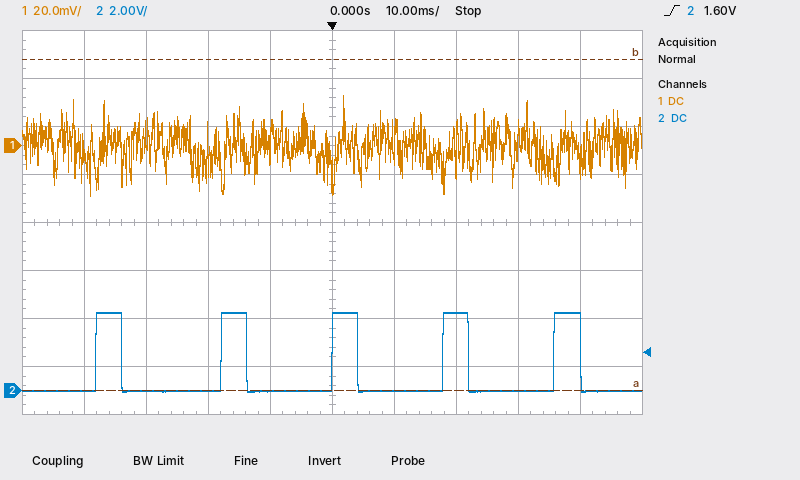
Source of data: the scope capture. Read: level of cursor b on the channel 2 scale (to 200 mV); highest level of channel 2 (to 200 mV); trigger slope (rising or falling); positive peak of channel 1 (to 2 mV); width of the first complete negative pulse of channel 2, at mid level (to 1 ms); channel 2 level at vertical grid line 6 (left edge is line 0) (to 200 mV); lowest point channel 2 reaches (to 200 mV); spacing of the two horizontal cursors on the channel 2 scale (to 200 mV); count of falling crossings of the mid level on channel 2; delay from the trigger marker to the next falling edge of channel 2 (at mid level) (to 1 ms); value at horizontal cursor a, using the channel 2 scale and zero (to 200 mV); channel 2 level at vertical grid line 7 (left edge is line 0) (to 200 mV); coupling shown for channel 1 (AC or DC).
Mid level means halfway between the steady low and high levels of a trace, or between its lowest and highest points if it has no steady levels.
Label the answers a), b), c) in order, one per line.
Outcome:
a) 13.8 V
b) 3.2 V
c) rising
d) 20 mV
e) 16 ms
f) 0.0 V
g) 0.0 V
h) 13.8 V
i) 5
j) 4 ms
k) 0.0 V
l) 3.2 V
m) DC
